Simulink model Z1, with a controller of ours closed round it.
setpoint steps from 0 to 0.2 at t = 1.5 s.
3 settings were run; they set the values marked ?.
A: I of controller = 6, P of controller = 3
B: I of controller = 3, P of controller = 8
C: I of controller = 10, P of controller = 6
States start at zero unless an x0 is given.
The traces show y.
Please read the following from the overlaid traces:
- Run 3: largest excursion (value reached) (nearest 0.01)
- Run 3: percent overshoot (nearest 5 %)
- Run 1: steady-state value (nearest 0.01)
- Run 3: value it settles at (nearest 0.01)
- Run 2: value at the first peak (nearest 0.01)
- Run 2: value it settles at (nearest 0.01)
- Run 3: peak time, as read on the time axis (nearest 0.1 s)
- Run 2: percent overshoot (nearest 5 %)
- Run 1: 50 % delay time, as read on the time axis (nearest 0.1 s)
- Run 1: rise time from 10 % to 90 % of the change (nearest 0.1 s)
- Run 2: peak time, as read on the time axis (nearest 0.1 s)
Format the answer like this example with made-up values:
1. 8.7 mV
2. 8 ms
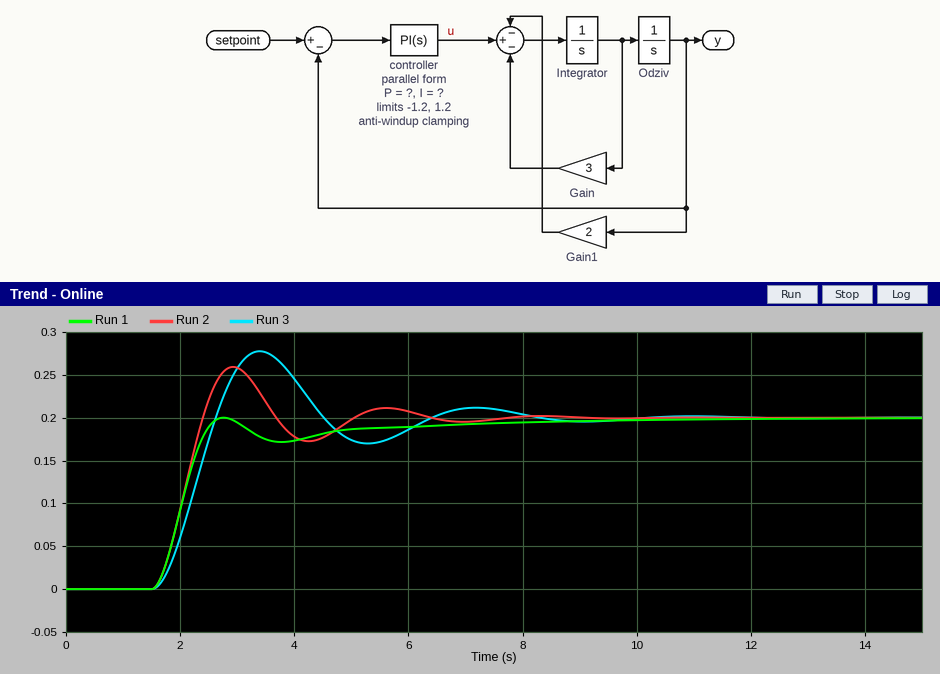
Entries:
1. 0.28
2. 40 %
3. 0.20
4. 0.20
5. 0.26
6. 0.20
7. 3.4 s
8. 30 %
9. 2.0 s
10. 0.7 s
11. 2.9 s
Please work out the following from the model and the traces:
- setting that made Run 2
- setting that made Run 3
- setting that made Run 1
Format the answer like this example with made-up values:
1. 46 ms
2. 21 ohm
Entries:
1. C
2. A
3. B
